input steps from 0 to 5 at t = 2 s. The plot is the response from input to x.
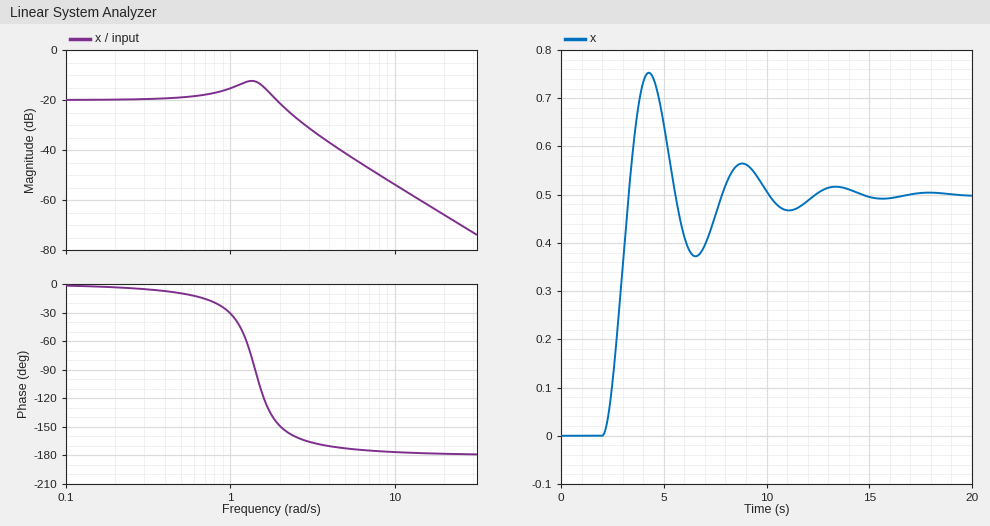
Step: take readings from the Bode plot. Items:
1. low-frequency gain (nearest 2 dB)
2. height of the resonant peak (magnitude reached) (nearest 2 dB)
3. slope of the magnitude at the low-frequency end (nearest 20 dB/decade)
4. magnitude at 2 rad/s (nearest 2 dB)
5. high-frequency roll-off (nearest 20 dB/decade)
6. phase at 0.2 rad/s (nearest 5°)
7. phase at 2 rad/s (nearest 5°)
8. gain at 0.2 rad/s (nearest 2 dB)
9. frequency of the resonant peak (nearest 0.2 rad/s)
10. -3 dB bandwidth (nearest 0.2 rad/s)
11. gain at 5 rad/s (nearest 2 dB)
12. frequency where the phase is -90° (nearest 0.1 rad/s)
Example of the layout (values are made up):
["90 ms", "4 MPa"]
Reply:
["-20 dB", "-12 dB", "0 dB/decade", "-22 dB", "-40 dB/decade", "-5°", "-150°", "-20 dB", "1.4 rad/s", "2.2 rad/s", "-42 dB", "1.4 rad/s"]
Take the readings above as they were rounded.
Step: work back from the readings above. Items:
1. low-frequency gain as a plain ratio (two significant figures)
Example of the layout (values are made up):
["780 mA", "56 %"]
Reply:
["0.10"]
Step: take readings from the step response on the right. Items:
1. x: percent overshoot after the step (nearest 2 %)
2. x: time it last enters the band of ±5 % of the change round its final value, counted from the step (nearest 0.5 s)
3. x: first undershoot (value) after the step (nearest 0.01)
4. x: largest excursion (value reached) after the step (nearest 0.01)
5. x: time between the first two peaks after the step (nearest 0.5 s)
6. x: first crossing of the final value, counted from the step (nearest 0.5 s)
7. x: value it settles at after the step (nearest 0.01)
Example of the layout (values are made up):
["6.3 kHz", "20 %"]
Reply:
["50 %", "9.5 s", "0.37", "0.75", "4.5 s", "1.5 s", "0.50"]
